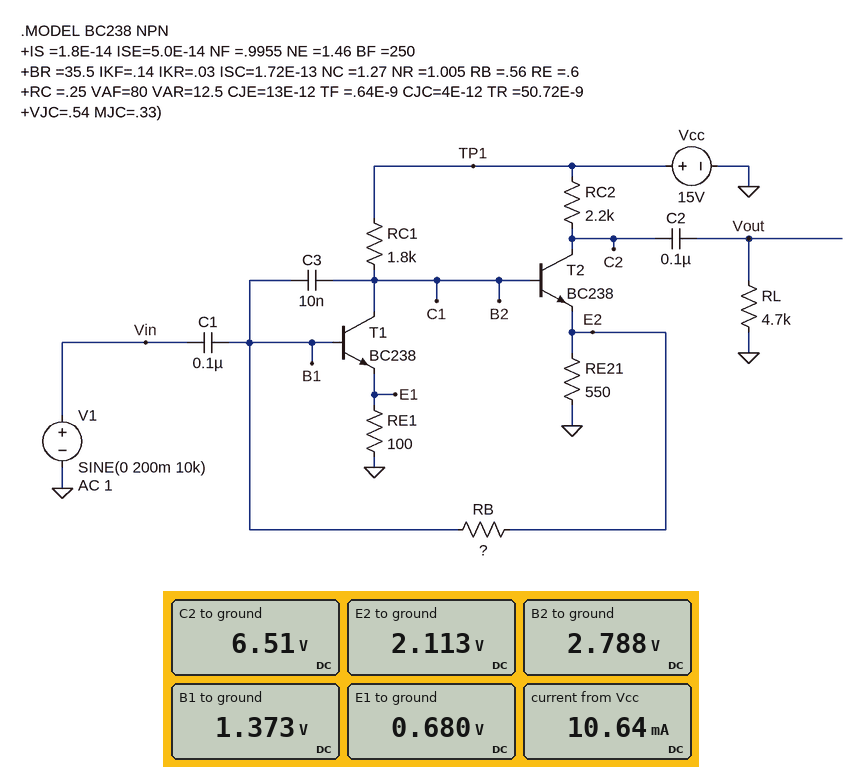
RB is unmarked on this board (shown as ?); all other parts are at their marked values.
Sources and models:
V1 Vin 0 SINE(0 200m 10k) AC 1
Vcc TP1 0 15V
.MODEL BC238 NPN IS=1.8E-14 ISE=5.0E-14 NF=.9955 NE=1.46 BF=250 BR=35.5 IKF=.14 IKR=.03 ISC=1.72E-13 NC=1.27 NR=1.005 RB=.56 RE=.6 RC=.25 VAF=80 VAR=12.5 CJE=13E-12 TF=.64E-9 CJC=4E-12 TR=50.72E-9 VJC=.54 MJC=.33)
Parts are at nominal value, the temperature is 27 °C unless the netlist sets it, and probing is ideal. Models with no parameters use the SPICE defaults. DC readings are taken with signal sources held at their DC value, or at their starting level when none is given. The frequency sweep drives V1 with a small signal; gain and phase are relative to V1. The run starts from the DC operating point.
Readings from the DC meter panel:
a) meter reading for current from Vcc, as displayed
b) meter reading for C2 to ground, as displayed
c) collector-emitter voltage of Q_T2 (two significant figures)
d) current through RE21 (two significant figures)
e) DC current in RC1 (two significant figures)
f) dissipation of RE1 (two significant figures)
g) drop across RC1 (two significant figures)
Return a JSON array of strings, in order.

["10.64 mA", "6.51 V", "4.4 V", "3.8 mA", "6.8 mA", "4.6 mW", "12 V"]
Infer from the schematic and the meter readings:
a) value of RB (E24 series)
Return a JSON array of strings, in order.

["22 kΩ"]
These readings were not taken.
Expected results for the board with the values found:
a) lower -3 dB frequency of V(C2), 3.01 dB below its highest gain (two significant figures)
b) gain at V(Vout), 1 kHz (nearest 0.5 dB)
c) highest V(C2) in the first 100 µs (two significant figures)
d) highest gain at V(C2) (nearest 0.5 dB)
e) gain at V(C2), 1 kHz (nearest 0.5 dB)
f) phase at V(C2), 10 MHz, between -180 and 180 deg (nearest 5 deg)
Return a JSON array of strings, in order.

["380 Hz", "23.5 dB", "9.5 V", "24.5 dB", "24.0 dB", "165 deg"]
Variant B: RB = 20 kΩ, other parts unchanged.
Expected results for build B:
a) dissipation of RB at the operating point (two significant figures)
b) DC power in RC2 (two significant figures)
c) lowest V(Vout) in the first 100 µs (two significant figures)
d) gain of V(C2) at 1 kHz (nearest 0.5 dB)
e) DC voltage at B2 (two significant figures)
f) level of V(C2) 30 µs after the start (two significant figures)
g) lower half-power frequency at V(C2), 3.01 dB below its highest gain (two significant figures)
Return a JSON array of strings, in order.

["23 µW", "31 mW", "-3.3 V", "23.5 dB", "2.7 V", "9.7 V", "430 Hz"]
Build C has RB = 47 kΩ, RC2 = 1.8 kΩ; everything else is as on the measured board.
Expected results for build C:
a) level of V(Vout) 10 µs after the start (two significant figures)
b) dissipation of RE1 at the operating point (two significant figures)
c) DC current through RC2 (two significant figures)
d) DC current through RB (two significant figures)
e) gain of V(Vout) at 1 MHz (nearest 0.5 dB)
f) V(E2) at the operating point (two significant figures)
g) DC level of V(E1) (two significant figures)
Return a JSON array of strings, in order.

["710 mV", "4.1 mW", "5.1 mA", "31 µA", "7.5 dB", "2.8 V", "640 mV"]
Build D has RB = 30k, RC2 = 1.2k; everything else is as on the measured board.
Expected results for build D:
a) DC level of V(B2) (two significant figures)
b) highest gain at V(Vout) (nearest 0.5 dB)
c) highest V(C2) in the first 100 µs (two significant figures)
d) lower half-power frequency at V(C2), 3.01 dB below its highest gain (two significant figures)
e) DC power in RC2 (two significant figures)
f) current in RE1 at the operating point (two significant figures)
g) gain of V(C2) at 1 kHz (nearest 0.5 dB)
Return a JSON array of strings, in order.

["3.0 V", "20.5 dB", "12 V", "290 Hz", "22 mW", "6.7 mA", "20.0 dB"]
